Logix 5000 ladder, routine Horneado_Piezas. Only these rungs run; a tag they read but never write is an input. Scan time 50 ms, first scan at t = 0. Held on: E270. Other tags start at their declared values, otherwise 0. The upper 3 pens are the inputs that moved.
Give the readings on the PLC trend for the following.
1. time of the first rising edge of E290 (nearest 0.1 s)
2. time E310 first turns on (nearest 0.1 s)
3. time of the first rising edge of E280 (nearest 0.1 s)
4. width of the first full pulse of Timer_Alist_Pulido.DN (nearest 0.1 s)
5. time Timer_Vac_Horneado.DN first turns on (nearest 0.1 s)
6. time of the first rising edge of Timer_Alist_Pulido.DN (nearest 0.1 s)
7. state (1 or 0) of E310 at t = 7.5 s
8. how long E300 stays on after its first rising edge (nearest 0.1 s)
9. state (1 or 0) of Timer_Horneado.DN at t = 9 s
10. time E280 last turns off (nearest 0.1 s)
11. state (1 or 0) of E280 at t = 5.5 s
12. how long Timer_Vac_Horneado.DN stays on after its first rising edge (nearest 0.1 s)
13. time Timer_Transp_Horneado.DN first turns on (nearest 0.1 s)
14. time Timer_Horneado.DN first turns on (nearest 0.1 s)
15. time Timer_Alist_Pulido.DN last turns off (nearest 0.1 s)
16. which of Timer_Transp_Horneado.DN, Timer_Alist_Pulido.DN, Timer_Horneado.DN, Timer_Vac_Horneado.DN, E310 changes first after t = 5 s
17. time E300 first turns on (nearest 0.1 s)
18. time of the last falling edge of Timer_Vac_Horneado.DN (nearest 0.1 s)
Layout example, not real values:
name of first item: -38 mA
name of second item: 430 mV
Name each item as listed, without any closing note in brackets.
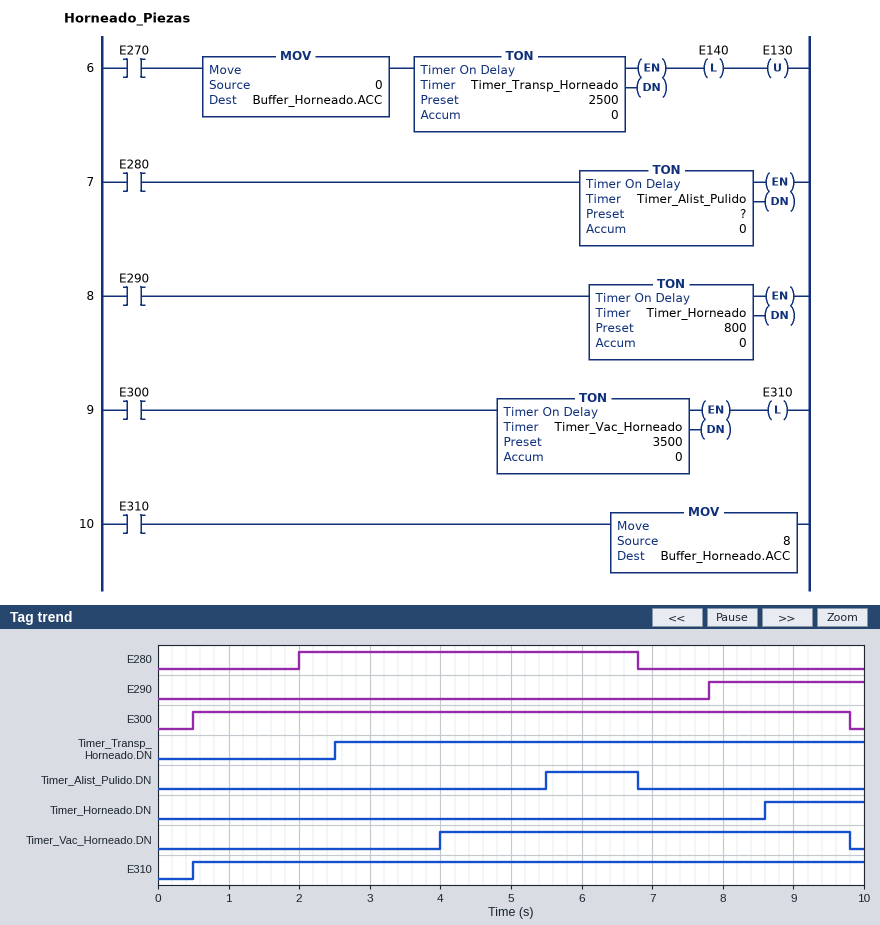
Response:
time of the first rising edge of E290: 7.8 s
time E310 first turns on: 0.5 s
time of the first rising edge of E280: 2.0 s
width of the first full pulse of Timer_Alist_Pulido.DN: 1.3 s
time Timer_Vac_Horneado.DN first turns on: 4.0 s
time of the first rising edge of Timer_Alist_Pulido.DN: 5.5 s
state (1 or 0) of E310 at t = 7.5 s: 1
how long E300 stays on after its first rising edge: 9.3 s
state (1 or 0) of Timer_Horneado.DN at t = 9 s: 1
time E280 last turns off: 6.8 s
state (1 or 0) of E280 at t = 5.5 s: 1
how long Timer_Vac_Horneado.DN stays on after its first rising edge: 5.8 s
time Timer_Transp_Horneado.DN first turns on: 2.5 s
time Timer_Horneado.DN first turns on: 8.6 s
time Timer_Alist_Pulido.DN last turns off: 6.8 s
which of Timer_Transp_Horneado.DN, Timer_Alist_Pulido.DN, Timer_Horneado.DN, Timer_Vac_Horneado.DN, E310 changes first after t = 5 s: Timer_Alist_Pulido.DN
time E300 first turns on: 0.5 s
time of the last falling edge of Timer_Vac_Horneado.DN: 9.8 s
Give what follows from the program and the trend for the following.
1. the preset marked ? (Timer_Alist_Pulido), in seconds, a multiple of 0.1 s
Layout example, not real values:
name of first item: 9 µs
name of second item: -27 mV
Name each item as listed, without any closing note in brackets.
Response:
the preset marked ? (Timer_Alist_Pulido), in seconds, a multiple of 0.1 s: 3.5 s
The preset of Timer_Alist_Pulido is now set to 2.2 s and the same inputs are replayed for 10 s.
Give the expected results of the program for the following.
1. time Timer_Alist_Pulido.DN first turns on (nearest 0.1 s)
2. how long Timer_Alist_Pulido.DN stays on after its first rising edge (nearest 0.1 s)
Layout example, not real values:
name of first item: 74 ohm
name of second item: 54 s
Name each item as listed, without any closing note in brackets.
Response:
time Timer_Alist_Pulido.DN first turns on: 4.2 s
how long Timer_Alist_Pulido.DN stays on after its first rising edge: 2.6 s
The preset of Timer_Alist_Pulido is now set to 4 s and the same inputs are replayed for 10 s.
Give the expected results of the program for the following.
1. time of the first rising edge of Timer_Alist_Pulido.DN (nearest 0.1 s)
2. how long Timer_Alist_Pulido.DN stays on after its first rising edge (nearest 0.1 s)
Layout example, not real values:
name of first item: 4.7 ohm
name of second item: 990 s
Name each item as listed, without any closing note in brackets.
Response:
time of the first rising edge of Timer_Alist_Pulido.DN: 6.0 s
how long Timer_Alist_Pulido.DN stays on after its first rising edge: 0.8 s
